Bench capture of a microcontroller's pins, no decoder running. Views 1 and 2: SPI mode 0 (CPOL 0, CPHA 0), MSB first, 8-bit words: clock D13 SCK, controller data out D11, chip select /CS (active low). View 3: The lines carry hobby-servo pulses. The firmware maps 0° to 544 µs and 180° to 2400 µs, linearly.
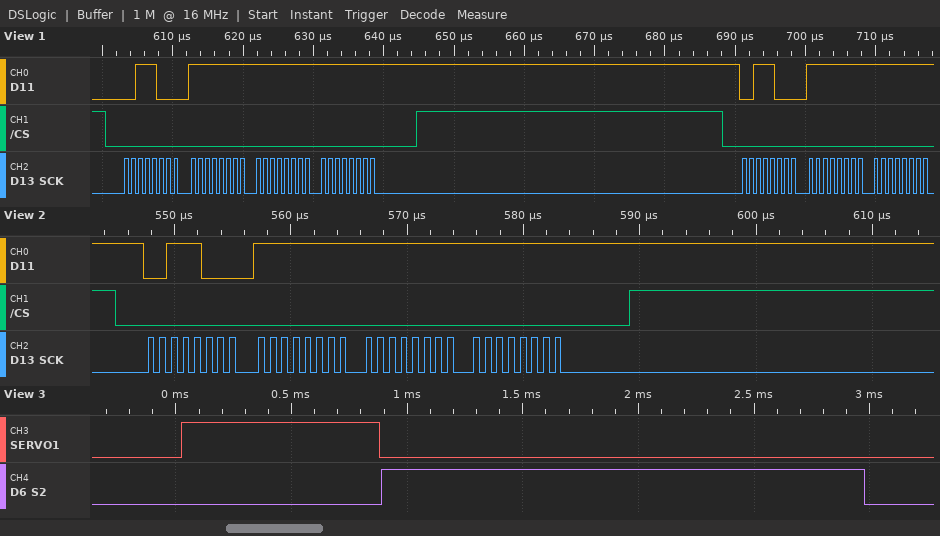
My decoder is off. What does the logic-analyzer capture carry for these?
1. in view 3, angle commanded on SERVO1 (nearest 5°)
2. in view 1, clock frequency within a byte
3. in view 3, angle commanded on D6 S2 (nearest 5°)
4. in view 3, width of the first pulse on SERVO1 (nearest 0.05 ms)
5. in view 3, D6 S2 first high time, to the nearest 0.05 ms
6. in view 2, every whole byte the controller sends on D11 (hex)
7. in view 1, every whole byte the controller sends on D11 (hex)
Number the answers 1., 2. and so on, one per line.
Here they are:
1. 30°
2. 1 MHz
3. 150°
4. 0.85 ms
5. 2.10 ms
6. 0x38 0xFF 0xFF 0xFF
7. 38 FF FF FF 38 FF FF
